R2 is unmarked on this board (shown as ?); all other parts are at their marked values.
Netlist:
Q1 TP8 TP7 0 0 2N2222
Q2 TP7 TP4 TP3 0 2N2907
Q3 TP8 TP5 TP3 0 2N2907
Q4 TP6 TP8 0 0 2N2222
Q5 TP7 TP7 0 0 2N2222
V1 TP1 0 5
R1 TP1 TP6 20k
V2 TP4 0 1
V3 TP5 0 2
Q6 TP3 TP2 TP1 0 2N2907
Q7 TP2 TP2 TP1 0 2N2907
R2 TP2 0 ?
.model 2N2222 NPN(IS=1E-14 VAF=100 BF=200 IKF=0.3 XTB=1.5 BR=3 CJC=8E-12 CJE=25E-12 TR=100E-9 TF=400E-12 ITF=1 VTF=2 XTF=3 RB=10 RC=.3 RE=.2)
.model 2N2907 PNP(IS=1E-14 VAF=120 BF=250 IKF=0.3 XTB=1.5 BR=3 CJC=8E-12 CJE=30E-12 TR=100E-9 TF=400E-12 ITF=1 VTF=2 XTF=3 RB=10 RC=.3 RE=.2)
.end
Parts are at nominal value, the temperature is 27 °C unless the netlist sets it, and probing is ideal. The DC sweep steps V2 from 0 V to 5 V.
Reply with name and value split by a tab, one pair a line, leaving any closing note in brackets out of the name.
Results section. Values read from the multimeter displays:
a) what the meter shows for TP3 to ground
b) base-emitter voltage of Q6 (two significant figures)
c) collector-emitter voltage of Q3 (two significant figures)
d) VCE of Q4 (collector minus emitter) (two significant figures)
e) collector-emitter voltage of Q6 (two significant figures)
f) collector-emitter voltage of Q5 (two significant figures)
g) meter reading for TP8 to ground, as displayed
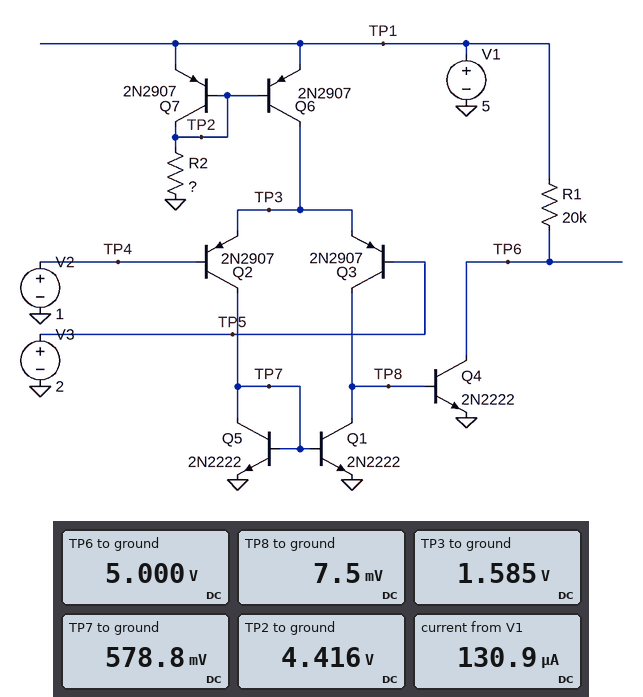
what the meter shows for TP3 to ground	1.585 V
base-emitter voltage of Q6	-580 mV
collector-emitter voltage of Q3	-1.6 V
VCE of Q4 (collector minus emitter)	5.0 V
collector-emitter voltage of Q6	-3.4 V
collector-emitter voltage of Q5	580 mV
meter reading for TP8 to ground, as displayed	7.5 mV
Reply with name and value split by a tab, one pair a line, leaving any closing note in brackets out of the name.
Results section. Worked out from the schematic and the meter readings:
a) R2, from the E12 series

R2, from the E12 series	68 kΩ
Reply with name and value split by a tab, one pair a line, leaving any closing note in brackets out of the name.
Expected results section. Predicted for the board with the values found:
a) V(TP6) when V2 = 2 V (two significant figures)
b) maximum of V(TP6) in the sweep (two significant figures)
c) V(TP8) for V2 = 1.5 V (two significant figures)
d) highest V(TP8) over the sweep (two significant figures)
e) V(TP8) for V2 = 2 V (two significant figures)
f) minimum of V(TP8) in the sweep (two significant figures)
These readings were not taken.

V(TP6) when V2 = 2 V	3.7 V
maximum of V(TP6) in the sweep	5.0 V
V(TP8) for V2 = 1.5 V	7.5 mV
highest V(TP8) over the sweep	640 mV
V(TP8) for V2 = 2 V	580 mV
minimum of V(TP8) in the sweep	7.5 mV
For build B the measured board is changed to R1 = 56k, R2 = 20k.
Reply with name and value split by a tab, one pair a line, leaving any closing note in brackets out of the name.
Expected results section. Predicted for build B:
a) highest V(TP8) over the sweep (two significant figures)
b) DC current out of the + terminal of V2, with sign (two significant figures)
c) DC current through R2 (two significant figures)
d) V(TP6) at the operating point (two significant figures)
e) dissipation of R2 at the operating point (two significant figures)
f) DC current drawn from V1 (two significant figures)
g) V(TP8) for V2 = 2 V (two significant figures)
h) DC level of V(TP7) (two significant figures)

highest V(TP8) over the sweep	660 mV
DC current out of the + terminal of V2, with sign	-880 nA
DC current through R2	220 µA
V(TP6) at the operating point	5.0 V
dissipation of R2 at the operating point	960 µW
DC current drawn from V1	440 µA
V(TP8) for V2 = 2 V	590 mV
DC level of V(TP7)	610 mV
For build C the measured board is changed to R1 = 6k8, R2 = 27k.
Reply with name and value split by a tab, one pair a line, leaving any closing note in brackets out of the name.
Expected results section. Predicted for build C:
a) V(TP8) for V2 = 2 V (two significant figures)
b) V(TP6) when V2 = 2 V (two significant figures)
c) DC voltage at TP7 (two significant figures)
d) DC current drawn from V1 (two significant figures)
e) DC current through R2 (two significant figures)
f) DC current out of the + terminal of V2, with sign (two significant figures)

V(TP8) for V2 = 2 V	610 mV
V(TP6) when V2 = 2 V	3.9 V
DC voltage at TP7	600 mV
DC current drawn from V1	330 µA
DC current through R2	160 µA
DC current out of the + terminal of V2, with sign	-660 nA
